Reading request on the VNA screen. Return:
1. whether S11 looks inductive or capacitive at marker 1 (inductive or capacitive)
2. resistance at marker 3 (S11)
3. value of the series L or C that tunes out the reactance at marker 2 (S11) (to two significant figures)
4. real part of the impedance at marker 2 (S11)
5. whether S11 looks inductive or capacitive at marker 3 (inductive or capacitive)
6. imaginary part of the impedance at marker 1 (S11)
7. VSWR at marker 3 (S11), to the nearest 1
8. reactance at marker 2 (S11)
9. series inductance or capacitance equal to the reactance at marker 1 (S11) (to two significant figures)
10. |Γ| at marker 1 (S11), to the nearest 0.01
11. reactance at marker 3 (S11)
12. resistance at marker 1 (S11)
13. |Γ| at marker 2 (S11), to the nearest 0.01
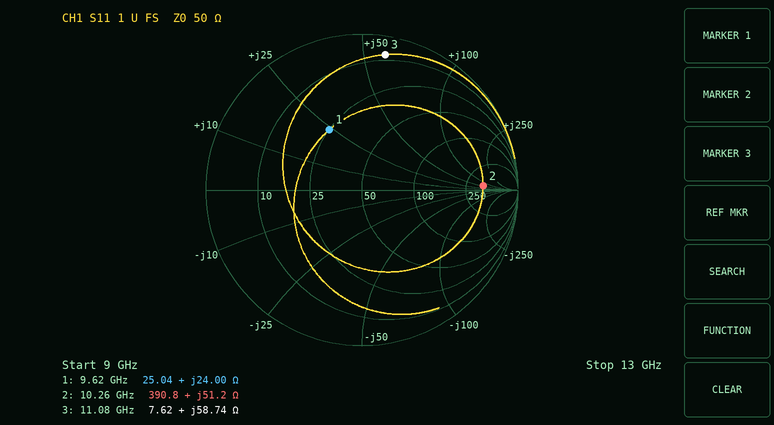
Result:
inductive
7.62 Ω
300 fF
390.8 Ω
inductive
+24.00 Ω
16
+51.2 Ω
400 pH
0.44
+58.74 Ω
25.04 Ω
0.78
